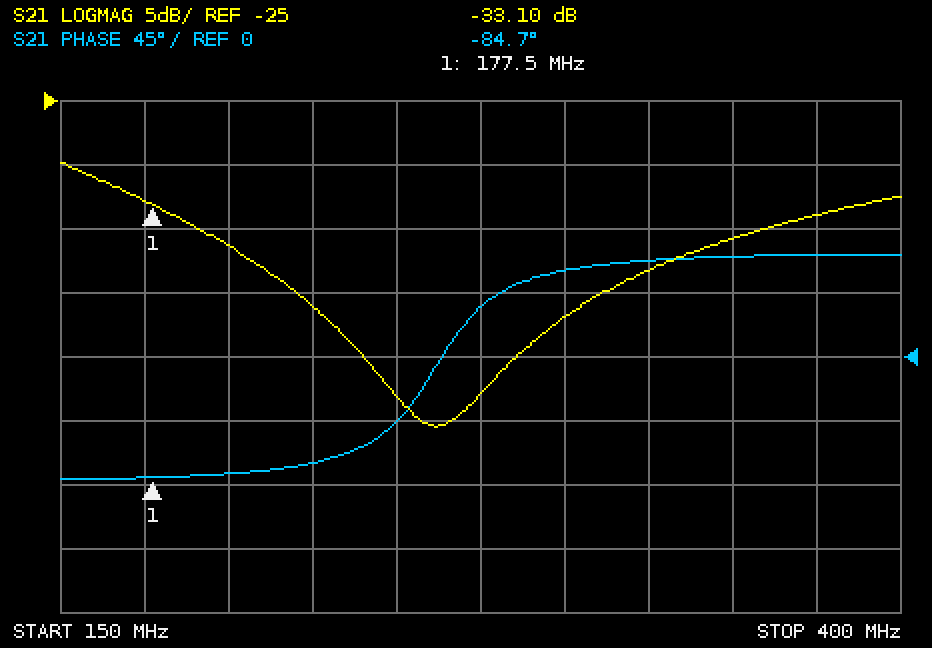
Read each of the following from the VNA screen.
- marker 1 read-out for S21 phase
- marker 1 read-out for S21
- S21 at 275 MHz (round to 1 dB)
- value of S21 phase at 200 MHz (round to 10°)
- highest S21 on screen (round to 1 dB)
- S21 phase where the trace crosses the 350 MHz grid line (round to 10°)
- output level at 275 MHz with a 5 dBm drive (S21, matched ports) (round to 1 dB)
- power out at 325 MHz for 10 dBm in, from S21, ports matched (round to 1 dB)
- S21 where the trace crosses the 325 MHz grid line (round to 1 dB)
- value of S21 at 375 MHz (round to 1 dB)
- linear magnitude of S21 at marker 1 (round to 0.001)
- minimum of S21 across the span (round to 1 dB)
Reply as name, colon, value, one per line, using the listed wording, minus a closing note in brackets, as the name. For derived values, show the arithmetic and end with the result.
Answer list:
marker 1 read-out for S21 phase: -84.7°
marker 1 read-out for S21: -33.10 dB
S21 at 275 MHz: -48 dB
value of S21 phase at 200 MHz: -80°
highest S21 on screen: -30 dB
S21 phase where the trace crosses the 350 MHz grid line: 70°
output level at 275 MHz with a 5 dBm drive (S21, matched ports): 5 dBm + (-48 dB) = -43 dBm
power out at 325 MHz for 10 dBm in, from S21, ports matched: 10 dBm + (-38 dB) = -28 dBm
S21 where the trace crosses the 325 MHz grid line: -38 dB
value of S21 at 375 MHz: -34 dB
linear magnitude of S21 at marker 1: 10^(-33.1/20) ≈ 0.022
minimum of S21 across the span: -50 dB
